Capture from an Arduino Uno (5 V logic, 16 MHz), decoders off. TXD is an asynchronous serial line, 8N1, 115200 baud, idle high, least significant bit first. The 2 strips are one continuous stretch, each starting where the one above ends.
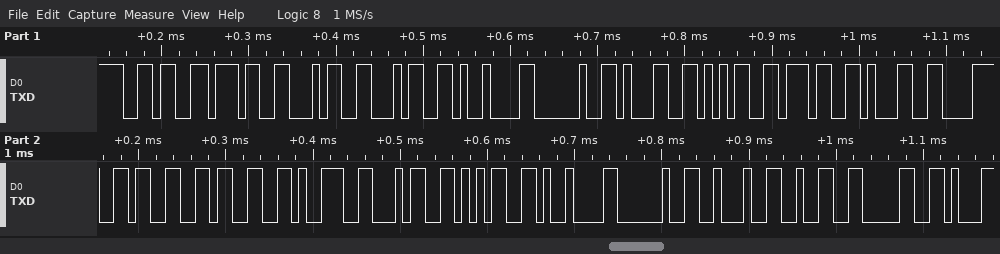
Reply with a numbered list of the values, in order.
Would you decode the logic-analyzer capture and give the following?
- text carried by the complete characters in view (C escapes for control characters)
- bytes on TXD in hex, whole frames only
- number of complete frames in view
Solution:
1. "6744\t 1571833945\t \"20"
2. 36 37 34 34 09 20 31 35 37 31 38 33 33 39 34 35 09 20 22 32 30
3. 21
